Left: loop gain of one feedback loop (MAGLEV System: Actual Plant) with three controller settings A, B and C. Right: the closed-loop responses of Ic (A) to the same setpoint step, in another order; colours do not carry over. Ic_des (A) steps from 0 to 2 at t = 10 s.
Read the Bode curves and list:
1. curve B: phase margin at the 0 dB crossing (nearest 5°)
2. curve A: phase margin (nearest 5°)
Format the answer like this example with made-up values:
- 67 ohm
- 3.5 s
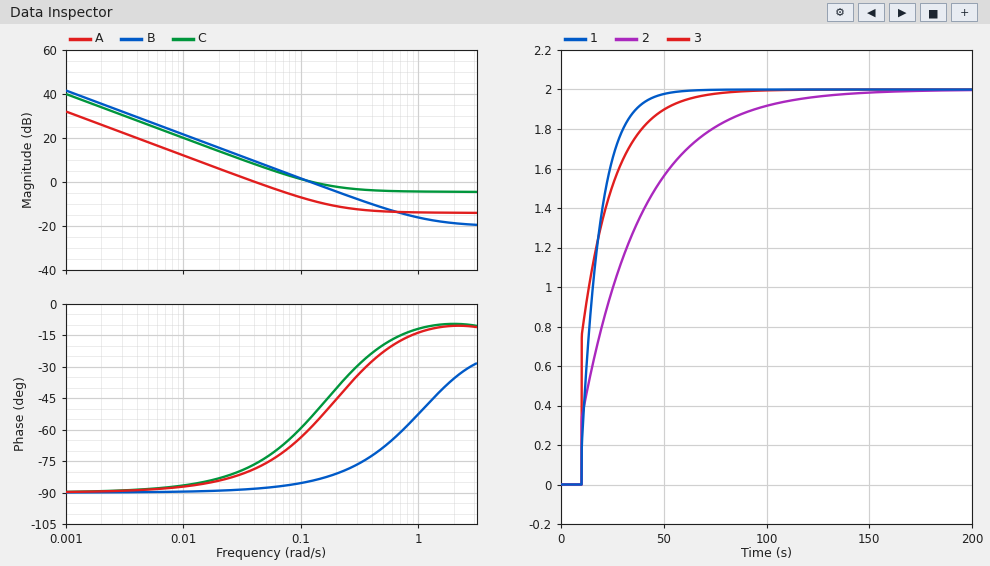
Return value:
- 95°
- 100°
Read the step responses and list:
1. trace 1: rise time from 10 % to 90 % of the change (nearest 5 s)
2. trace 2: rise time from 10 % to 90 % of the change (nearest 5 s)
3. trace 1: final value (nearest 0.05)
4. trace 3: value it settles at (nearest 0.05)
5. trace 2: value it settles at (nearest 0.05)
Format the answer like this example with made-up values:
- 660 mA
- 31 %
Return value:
- 20 s
- 65 s
- 2.00
- 2.00
- 2.00
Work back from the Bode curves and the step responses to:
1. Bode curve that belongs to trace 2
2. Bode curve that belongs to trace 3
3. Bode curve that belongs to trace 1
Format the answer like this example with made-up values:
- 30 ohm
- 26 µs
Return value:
- A
- C
- B
